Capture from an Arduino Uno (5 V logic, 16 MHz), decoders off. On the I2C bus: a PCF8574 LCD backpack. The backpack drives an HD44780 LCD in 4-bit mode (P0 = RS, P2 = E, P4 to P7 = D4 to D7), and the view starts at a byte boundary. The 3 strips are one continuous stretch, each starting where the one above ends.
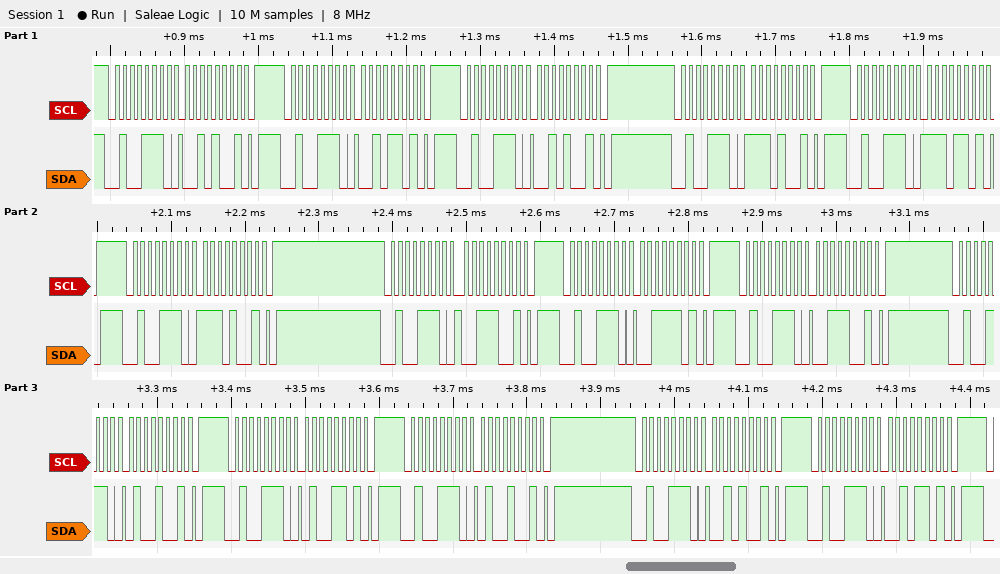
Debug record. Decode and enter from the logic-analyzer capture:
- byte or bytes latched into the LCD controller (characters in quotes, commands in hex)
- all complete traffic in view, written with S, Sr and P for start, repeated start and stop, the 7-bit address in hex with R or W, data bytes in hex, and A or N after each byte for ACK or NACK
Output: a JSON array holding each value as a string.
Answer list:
["'.' '4'", "S 27W A 29 A P S 27W A 2D A P S 27W A 29 A P S 27W A E9 A P S 27W A ED A P S 27W A E9 A P S 27W A 39 A P S 27W A 3D A P S 27W A 39 A P S 27W A 49 A P S 27W A 4D A P S 27W A 49 A P S 27W A 29 A P S 27W A 2D A P"]
